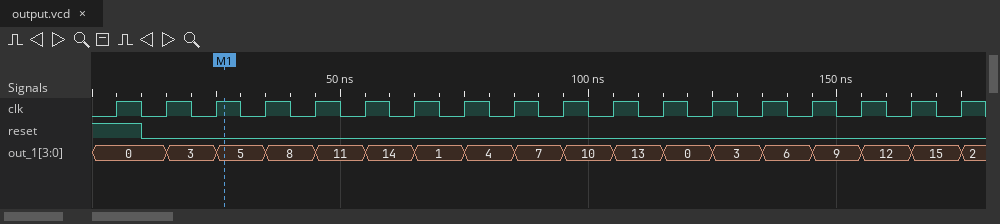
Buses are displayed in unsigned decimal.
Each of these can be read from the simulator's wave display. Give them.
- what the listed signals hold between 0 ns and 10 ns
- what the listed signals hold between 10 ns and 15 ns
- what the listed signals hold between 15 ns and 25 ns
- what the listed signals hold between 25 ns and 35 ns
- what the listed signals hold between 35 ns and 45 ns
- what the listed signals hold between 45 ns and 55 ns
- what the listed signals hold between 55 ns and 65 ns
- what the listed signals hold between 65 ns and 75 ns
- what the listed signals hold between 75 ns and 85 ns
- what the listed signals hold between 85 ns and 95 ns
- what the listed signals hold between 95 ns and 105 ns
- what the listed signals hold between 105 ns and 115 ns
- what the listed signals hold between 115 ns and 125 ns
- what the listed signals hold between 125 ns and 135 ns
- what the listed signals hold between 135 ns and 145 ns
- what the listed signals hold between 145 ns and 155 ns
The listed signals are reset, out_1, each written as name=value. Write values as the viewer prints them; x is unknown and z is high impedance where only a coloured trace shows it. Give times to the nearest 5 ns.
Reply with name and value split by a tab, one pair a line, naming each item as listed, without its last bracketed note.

what the listed signals hold between 0 ns and 10 ns	reset=1, out_1=0
what the listed signals hold between 10 ns and 15 ns	reset=0, out_1=0
what the listed signals hold between 15 ns and 25 ns	reset=0, out_1=3
what the listed signals hold between 25 ns and 35 ns	reset=0, out_1=5
what the listed signals hold between 35 ns and 45 ns	reset=0, out_1=8
what the listed signals hold between 45 ns and 55 ns	reset=0, out_1=11
what the listed signals hold between 55 ns and 65 ns	reset=0, out_1=14
what the listed signals hold between 65 ns and 75 ns	reset=0, out_1=1
what the listed signals hold between 75 ns and 85 ns	reset=0, out_1=4
what the listed signals hold between 85 ns and 95 ns	reset=0, out_1=7
what the listed signals hold between 95 ns and 105 ns	reset=0, out_1=10
what the listed signals hold between 105 ns and 115 ns	reset=0, out_1=13
what the listed signals hold between 115 ns and 125 ns	reset=0, out_1=0
what the listed signals hold between 125 ns and 135 ns	reset=0, out_1=3
what the listed signals hold between 135 ns and 145 ns	reset=0, out_1=6
what the listed signals hold between 145 ns and 155 ns	reset=0, out_1=9
